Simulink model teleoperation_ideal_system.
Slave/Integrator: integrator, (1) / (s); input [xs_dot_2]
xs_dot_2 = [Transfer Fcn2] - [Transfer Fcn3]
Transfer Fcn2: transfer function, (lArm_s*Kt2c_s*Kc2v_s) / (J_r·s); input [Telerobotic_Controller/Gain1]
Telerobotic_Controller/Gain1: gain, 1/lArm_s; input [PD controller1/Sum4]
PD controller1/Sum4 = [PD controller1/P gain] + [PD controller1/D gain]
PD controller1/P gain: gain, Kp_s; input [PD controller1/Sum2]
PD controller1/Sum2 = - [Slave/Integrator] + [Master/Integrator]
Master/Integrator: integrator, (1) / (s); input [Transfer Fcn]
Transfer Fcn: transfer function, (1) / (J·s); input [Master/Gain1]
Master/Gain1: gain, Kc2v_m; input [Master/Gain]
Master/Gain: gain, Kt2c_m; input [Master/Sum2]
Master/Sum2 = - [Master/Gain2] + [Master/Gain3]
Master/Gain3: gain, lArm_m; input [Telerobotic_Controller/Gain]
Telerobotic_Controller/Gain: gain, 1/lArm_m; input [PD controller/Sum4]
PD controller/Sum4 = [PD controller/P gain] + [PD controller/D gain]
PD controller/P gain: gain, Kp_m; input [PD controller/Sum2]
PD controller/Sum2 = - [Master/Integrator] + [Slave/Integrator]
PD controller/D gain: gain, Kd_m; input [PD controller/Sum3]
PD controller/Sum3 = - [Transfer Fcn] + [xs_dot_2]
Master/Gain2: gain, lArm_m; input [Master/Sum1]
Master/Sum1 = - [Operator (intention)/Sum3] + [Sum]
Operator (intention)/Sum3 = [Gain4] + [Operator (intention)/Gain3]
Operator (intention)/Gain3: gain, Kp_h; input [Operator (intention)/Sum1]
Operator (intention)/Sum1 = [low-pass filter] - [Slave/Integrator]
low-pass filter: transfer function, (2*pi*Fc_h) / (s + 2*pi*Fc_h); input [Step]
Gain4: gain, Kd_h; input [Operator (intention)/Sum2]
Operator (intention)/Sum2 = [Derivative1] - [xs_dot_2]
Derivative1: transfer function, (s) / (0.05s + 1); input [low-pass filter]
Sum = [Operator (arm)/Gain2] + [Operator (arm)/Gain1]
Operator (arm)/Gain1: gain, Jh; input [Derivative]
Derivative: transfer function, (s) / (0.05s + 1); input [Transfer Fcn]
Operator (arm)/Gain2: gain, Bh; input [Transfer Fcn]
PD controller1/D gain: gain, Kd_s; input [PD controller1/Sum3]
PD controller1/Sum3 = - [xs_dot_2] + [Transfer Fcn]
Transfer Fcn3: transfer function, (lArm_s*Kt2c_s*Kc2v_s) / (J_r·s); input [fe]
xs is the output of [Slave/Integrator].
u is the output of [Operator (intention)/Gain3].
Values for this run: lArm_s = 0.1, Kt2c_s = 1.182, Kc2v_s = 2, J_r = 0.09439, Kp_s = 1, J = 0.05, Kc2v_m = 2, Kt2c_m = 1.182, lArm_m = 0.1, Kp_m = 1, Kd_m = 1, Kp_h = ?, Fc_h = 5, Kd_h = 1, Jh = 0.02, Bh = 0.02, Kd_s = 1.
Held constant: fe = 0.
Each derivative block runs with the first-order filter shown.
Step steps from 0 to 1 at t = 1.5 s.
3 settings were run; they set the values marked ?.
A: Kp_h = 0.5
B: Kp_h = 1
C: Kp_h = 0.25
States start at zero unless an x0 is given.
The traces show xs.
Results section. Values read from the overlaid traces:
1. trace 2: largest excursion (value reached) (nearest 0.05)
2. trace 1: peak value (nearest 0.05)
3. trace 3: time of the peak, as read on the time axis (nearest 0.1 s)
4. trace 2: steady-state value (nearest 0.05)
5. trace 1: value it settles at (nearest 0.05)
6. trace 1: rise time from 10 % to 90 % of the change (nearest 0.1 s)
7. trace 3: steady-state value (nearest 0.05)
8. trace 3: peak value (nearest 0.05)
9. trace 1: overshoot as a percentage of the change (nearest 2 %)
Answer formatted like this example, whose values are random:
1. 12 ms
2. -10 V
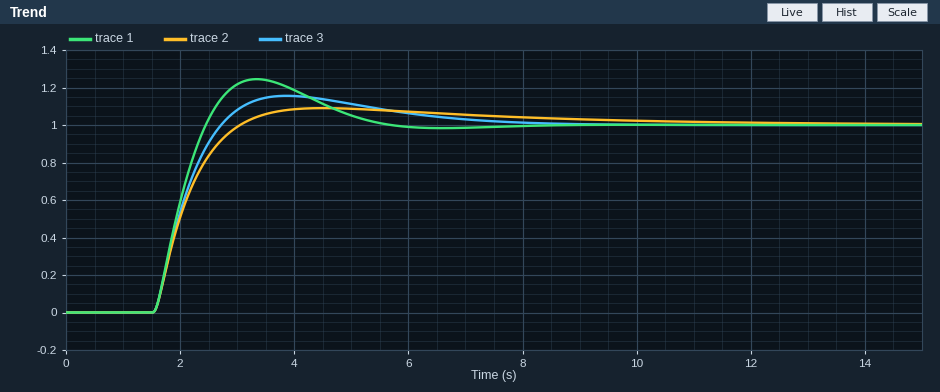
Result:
1. 1.10
2. 1.25
3. 3.9 s
4. 1.00
5. 1.00
6. 0.7 s
7. 1.00
8. 1.15
9. 24 %
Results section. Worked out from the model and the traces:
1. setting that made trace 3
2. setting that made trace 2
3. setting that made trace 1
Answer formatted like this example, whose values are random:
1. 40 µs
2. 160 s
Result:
1. A
2. C
3. B
